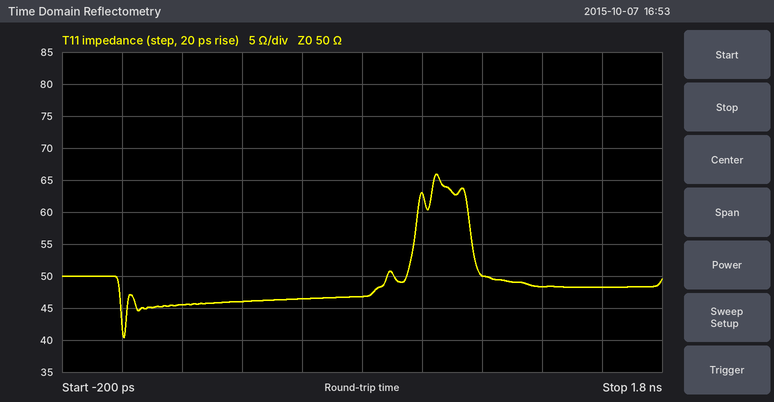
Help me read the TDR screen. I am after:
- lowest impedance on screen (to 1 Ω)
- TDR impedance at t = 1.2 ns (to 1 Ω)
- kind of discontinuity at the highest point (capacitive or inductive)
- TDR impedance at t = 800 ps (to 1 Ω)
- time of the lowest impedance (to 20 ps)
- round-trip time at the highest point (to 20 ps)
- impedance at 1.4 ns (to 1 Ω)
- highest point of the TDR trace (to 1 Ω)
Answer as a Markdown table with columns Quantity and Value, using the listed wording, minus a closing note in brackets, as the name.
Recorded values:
| Quantity | Value |
|---|---|
| lowest impedance on screen | 40 Ω |
| TDR impedance at t = 1.2 ns | 50 Ω |
| kind of discontinuity at the highest point | inductive |
| TDR impedance at t = 800 ps | 47 Ω |
| time of the lowest impedance | 0 ps |
| round-trip time at the highest point | 1.04 ns |
| impedance at 1.4 ns | 48 Ω |
| highest point of the TDR trace | 66 Ω |
